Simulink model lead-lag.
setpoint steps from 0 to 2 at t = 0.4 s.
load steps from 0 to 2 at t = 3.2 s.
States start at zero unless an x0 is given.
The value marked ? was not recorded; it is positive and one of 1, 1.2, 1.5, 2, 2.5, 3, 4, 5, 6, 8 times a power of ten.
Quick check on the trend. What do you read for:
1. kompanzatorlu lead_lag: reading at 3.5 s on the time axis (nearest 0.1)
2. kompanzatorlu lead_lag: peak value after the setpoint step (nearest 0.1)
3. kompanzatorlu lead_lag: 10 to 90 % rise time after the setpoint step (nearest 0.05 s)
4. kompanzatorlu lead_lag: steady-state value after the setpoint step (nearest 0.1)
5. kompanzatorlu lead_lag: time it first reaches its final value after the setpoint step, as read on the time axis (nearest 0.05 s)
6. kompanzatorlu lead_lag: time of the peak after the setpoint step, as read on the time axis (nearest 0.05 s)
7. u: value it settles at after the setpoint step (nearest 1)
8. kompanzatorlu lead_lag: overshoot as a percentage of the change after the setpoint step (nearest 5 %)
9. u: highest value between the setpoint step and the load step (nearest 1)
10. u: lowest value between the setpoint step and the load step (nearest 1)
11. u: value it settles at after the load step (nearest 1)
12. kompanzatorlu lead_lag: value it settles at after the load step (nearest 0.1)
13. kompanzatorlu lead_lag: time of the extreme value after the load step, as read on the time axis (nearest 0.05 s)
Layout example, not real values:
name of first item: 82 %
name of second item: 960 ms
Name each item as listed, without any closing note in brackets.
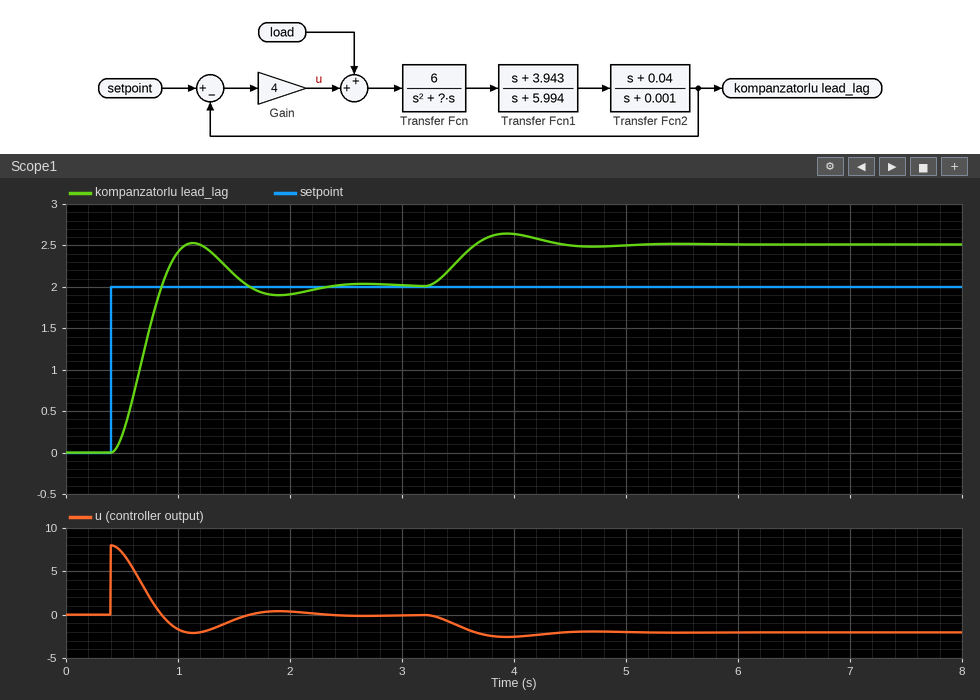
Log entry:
kompanzatorlu lead_lag: reading at 3.5 s on the time axis: 2.3
kompanzatorlu lead_lag: peak value after the setpoint step: 2.5
kompanzatorlu lead_lag: 10 to 90 % rise time after the setpoint step: 0.30 s
kompanzatorlu lead_lag: steady-state value after the setpoint step: 2.0
kompanzatorlu lead_lag: time it first reaches its final value after the setpoint step, as read on the time axis: 0.85 s
kompanzatorlu lead_lag: time of the peak after the setpoint step, as read on the time axis: 1.15 s
u: value it settles at after the setpoint step: 0
kompanzatorlu lead_lag: overshoot as a percentage of the change after the setpoint step: 25 %
u: highest value between the setpoint step and the load step: 8
u: lowest value between the setpoint step and the load step: -2
u: value it settles at after the load step: -2
kompanzatorlu lead_lag: value it settles at after the load step: 2.5
kompanzatorlu lead_lag: time of the extreme value after the load step, as read on the time axis: 3.95 s
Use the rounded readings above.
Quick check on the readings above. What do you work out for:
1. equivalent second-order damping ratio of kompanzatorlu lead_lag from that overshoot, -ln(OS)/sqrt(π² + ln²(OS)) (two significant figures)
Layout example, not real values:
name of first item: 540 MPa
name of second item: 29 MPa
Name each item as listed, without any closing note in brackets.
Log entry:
equivalent second-order damping ratio of kompanzatorlu lead_lag from that overshoot, -ln(OS)/sqrt(π² + ln²(OS)): 0.40
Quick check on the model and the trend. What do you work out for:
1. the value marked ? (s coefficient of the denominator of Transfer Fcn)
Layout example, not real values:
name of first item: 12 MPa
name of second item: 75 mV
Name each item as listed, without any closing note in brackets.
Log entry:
the value marked ?: 2.5
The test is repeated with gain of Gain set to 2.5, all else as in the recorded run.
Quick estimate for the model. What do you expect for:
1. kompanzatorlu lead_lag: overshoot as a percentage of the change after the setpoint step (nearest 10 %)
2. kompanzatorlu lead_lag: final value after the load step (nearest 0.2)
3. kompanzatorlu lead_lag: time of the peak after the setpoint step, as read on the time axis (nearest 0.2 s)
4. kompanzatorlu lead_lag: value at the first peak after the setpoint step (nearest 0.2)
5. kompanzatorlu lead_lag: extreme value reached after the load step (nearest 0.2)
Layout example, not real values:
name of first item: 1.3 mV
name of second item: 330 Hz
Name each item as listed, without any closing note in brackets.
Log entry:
kompanzatorlu lead_lag: overshoot as a percentage of the change after the setpoint step: 20 %
kompanzatorlu lead_lag: final value after the load step: 2.8
kompanzatorlu lead_lag: time of the peak after the setpoint step, as read on the time axis: 1.4 s
kompanzatorlu lead_lag: value at the first peak after the setpoint step: 2.4
kompanzatorlu lead_lag: extreme value reached after the load step: 3.0
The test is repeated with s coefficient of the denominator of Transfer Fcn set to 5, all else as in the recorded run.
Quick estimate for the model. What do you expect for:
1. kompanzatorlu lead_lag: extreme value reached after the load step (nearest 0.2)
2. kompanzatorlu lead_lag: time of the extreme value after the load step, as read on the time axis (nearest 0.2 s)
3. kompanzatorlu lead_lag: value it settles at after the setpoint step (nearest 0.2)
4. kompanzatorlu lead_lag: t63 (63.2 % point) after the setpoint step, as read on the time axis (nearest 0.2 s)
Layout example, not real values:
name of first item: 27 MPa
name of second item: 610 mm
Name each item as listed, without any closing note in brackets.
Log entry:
kompanzatorlu lead_lag: extreme value reached after the load step: 2.6
kompanzatorlu lead_lag: time of the extreme value after the load step, as read on the time axis: 4.2 s
kompanzatorlu lead_lag: value it settles at after the setpoint step: 2.0
kompanzatorlu lead_lag: t63 (63.2 % point) after the setpoint step, as read on the time axis: 0.8 s
